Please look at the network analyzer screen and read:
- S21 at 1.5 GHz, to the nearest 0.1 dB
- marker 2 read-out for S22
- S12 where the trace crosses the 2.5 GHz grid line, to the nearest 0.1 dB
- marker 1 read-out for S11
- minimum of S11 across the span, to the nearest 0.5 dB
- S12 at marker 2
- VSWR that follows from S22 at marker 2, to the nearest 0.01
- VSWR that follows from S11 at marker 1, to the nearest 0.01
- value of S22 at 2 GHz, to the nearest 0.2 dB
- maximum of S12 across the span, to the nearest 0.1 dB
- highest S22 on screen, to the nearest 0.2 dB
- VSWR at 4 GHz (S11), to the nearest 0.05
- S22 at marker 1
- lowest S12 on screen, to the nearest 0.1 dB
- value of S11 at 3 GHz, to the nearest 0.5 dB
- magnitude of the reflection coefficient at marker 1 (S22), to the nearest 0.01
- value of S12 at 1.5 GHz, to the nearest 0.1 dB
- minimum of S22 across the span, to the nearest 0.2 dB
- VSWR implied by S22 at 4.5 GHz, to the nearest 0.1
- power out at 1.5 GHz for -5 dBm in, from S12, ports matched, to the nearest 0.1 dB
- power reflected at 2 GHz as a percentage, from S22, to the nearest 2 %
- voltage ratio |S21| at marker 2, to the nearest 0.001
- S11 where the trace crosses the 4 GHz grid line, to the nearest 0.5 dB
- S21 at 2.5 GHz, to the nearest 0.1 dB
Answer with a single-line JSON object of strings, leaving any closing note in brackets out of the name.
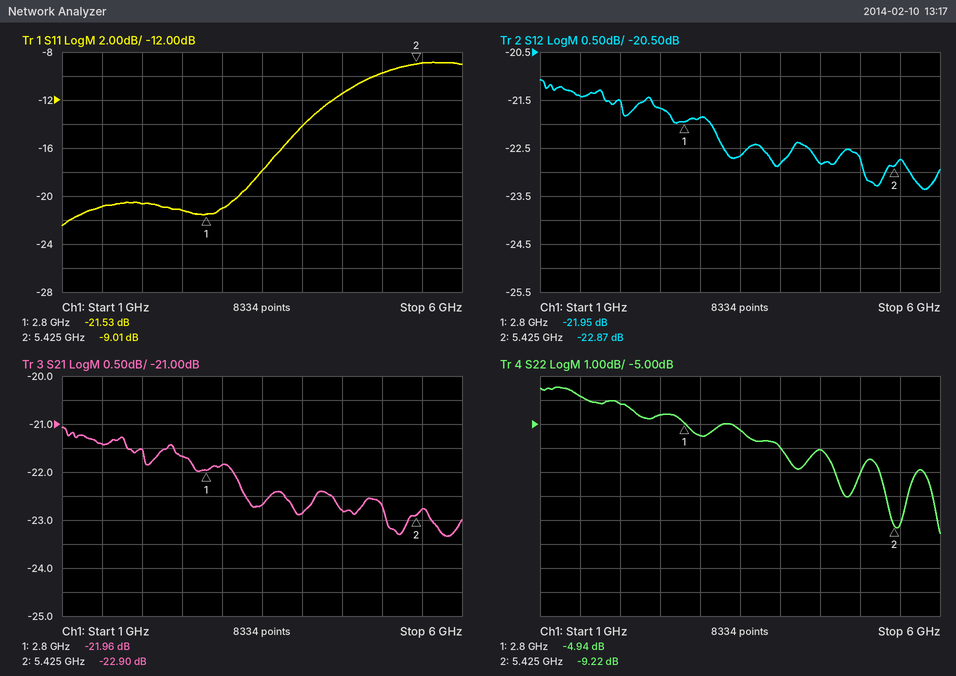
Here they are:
{"S21 at 1.5 GHz, to the nearest 0.1 dB": "-21.4 dB", "marker 2 read-out for S22": "-9.22 dB", "S12 where the trace crosses the 2.5 GHz grid line, to the nearest 0.1 dB": "-21.7 dB", "marker 1 read-out for S11": "-21.53 dB", "minimum of S11 across the span, to the nearest 0.5 dB": "-22.5 dB", "S12 at marker 2": "-22.87 dB", "VSWR that follows from S22 at marker 2, to the nearest 0.01": "2.06", "VSWR that follows from S11 at marker 1, to the nearest 0.01": "1.18", "value of S22 at 2 GHz, to the nearest 0.2 dB": "-4.2 dB", "maximum of S12 across the span, to the nearest 0.1 dB": "-21.1 dB", "highest S22 on screen, to the nearest 0.2 dB": "-3.4 dB", "VSWR at 4 GHz (S11), to the nearest 0.05": "1.50", "S22 at marker 1": "-4.94 dB", "lowest S12 on screen, to the nearest 0.1 dB": "-23.4 dB", "value of S11 at 3 GHz, to the nearest 0.5 dB": "-21.0 dB", "magnitude of the reflection coefficient at marker 1 (S22), to the nearest 0.01": "0.57", "value of S12 at 1.5 GHz, to the nearest 0.1 dB": "-21.4 dB", "minimum of S22 across the span, to the nearest 0.2 dB": "-9.6 dB", "VSWR implied by S22 at 4.5 GHz, to the nearest 0.1": "3.0", "power out at 1.5 GHz for -5 dBm in, from S12, ports matched, to the nearest 0.1 dB": "-26.4 dBm", "power reflected at 2 GHz as a percentage, from S22, to the nearest 2 %": "38 %", "voltage ratio |S21| at marker 2, to the nearest 0.001": "0.072", "S11 where the trace crosses the 4 GHz grid line, to the nearest 0.5 dB": "-14.0 dB", "S21 at 2.5 GHz, to the nearest 0.1 dB": "-21.7 dB"}
